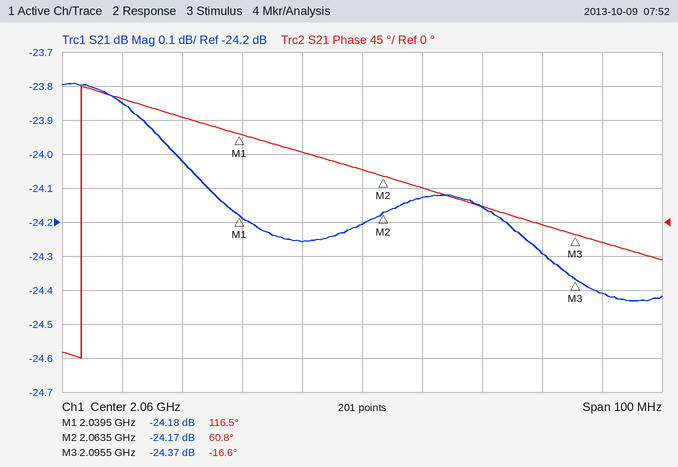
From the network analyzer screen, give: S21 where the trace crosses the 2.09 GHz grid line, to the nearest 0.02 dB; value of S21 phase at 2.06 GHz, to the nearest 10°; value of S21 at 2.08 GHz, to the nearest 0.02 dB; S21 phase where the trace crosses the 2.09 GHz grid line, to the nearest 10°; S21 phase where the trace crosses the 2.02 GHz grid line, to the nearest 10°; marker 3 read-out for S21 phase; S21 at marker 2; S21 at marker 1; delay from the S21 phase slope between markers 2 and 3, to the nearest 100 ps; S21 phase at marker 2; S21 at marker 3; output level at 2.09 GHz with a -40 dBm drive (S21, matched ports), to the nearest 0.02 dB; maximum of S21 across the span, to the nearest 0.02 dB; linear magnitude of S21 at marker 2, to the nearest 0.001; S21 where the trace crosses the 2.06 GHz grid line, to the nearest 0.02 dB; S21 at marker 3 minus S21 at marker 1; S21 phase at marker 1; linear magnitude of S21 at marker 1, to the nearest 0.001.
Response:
-24.30 dB
70°
-24.16 dB
0°
160°
-16.6°
-24.17 dB
-24.18 dB
6.7 ns
60.8°
-24.37 dB
-64.30 dBm
-23.80 dB
0.062
-24.20 dB
-0.19 dB
116.5°
0.062
